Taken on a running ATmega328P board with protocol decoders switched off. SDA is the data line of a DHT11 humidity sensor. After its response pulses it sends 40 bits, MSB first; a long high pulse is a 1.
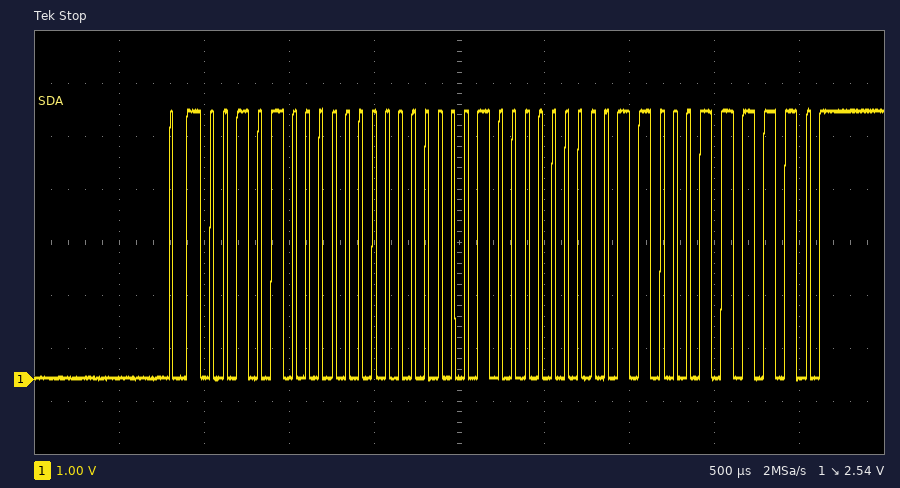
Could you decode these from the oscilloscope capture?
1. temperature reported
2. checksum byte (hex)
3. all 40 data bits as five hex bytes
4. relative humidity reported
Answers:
16.6 °C
0x3E
28 00 10 06 3E
40 %
